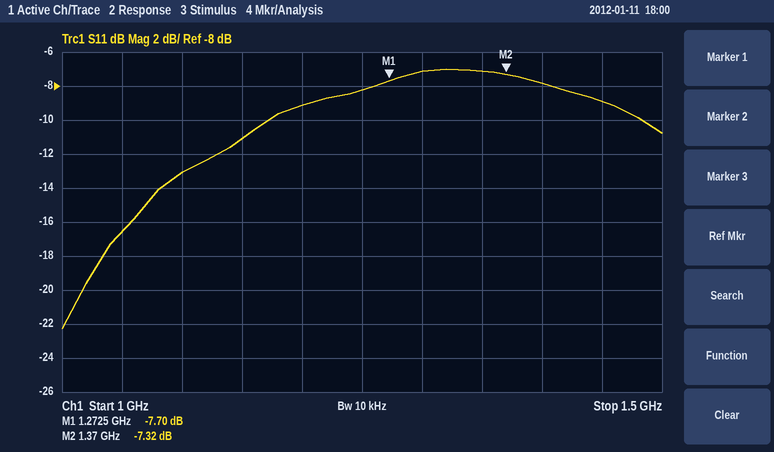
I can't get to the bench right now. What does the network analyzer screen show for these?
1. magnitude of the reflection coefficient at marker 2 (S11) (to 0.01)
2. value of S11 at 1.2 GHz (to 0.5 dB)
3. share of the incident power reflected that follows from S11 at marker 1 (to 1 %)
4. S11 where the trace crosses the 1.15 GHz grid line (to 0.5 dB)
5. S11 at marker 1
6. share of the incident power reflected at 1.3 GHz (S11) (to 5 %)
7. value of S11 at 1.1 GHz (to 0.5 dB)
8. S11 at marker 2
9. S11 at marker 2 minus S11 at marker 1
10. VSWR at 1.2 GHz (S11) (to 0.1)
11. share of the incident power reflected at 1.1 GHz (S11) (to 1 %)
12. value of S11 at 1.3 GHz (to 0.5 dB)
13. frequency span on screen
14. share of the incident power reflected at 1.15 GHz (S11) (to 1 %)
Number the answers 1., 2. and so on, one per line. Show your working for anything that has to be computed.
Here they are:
1. 10^(-7.32/20) ≈ 0.43
2. -9.0 dB
3. 10^(-7.7/10) ≈ 17 %
4. -11.0 dB
5. -7.70 dB
6. 10^(-7/10) ≈ 20 %
7. -13.0 dB
8. -7.32 dB
9. -7.32 − (-7.7) = 0.38 dB
10. |Γ| = 10^(-9/20) = 0.3548; VSWR = (1 + 0.3548)/(1 − 0.3548) ≈ 2.1
11. 10^(-13/10) ≈ 5 %
12. -7.0 dB
13. 500 MHz
14. 10^(-11/10) ≈ 8 %
